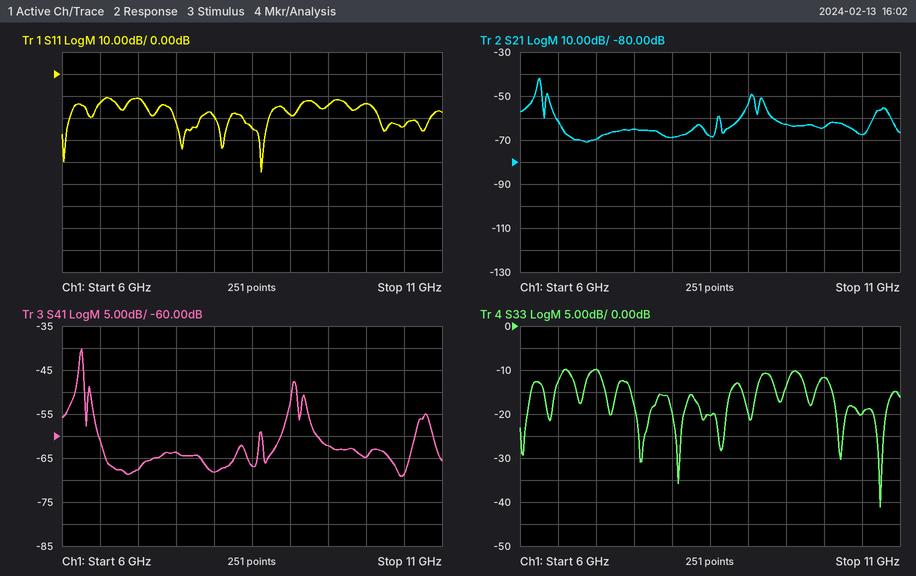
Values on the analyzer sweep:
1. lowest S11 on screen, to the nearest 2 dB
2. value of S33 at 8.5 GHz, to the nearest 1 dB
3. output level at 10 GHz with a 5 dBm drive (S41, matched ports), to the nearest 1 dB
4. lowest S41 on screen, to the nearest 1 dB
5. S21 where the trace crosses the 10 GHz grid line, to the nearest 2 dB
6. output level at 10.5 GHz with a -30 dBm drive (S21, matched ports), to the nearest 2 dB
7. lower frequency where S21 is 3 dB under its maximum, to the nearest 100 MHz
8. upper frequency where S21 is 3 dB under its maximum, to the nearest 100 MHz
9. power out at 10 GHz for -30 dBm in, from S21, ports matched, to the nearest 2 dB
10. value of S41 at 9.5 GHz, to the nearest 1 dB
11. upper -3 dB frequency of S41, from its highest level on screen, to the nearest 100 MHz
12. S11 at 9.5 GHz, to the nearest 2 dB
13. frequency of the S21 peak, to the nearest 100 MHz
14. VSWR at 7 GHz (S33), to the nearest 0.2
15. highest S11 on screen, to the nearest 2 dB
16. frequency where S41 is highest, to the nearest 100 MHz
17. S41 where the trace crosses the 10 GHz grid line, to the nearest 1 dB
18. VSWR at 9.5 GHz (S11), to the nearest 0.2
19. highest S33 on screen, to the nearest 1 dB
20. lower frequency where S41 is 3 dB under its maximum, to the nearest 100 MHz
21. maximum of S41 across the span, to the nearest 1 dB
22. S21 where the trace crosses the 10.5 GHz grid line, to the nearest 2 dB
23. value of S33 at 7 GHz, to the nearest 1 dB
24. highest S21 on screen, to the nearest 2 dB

-44 dB
-20 dB
-60 dBm
-69 dB
-64 dB
-98 dBm
6.2 GHz
6.3 GHz
-94 dBm
-62 dB
6.3 GHz
-14 dB
6.3 GHz
2.0
-10 dB
6.3 GHz
-65 dB
1.4
-10 dB
6.2 GHz
-40 dB
-68 dB
-10 dB
-42 dB
